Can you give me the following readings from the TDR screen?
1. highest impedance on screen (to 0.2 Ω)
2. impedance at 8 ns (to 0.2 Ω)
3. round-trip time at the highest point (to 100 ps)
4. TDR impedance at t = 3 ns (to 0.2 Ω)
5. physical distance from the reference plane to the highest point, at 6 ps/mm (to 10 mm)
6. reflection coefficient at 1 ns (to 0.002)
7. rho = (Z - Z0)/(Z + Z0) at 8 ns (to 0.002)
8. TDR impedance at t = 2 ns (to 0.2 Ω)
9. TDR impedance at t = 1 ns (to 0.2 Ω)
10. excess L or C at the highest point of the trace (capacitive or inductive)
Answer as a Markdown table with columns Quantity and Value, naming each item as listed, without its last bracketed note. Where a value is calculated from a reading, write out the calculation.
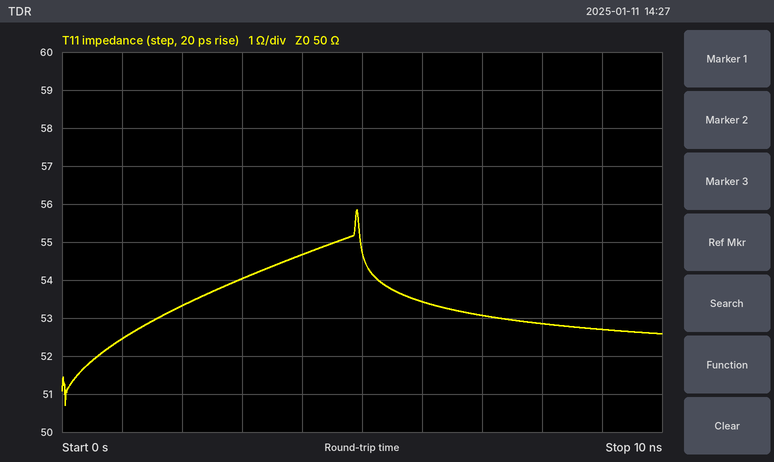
| Quantity | Value |
|---|---|
| highest impedance on screen | 55.8 Ω |
| impedance at 8 ns | 52.8 Ω |
| round-trip time at the highest point | 4.9 ns |
| TDR impedance at t = 3 ns | 54.0 Ω |
| physical distance from the reference plane to the highest point, at 6 ps/mm | 4.9 ns / 2 / 6 ps/mm ≈ 408 mm, so 410 mm to the nearest 10 mm |
| reflection coefficient at 1 ns | (52.4 − 50)/(52.4 + 50) ≈ +0.0234, so +0.024 to the nearest 0.002 |
| rho = (Z - Z0)/(Z + Z0) at 8 ns | (52.8 − 50)/(52.8 + 50) ≈ +0.0272, so +0.028 to the nearest 0.002 |
| TDR impedance at t = 2 ns | 53.4 Ω |
| TDR impedance at t = 1 ns | 52.4 Ω |
| excess L or C at the highest point of the trace | inductive |
